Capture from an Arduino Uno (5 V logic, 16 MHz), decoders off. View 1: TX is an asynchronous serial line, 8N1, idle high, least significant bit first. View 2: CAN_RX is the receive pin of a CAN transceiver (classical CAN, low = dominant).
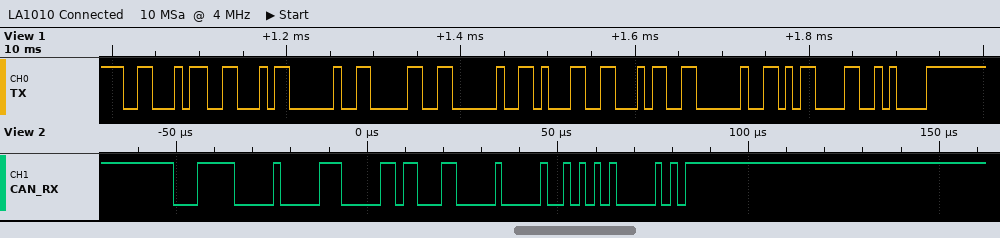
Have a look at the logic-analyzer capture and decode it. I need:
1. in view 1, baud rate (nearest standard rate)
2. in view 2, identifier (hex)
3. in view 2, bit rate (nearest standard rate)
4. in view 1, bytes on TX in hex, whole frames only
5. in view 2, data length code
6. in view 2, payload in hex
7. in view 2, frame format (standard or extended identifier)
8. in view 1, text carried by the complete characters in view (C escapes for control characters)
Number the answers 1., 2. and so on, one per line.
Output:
1. 115200 baud
2. 0x1F0
3. 500 kbit/s
4. 46 46 20 30 20 31 34 20 0D 0A
5. 3
6. 05 8C 00
7. standard
8. "FF 0 14 \r\n"
